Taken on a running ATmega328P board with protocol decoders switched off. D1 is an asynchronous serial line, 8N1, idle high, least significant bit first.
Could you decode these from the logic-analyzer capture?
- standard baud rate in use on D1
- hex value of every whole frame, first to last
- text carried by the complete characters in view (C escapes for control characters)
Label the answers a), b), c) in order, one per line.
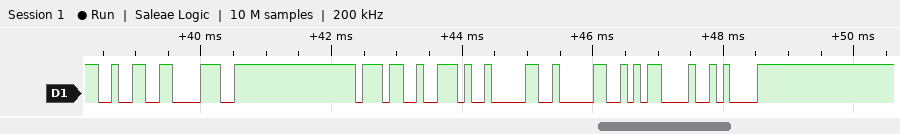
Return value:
a) 9600 baud
b) 0x32 0x38 0x37 0x2E 0x30 0x30 0x0D 0x0A
c) "287.00\r\n"
